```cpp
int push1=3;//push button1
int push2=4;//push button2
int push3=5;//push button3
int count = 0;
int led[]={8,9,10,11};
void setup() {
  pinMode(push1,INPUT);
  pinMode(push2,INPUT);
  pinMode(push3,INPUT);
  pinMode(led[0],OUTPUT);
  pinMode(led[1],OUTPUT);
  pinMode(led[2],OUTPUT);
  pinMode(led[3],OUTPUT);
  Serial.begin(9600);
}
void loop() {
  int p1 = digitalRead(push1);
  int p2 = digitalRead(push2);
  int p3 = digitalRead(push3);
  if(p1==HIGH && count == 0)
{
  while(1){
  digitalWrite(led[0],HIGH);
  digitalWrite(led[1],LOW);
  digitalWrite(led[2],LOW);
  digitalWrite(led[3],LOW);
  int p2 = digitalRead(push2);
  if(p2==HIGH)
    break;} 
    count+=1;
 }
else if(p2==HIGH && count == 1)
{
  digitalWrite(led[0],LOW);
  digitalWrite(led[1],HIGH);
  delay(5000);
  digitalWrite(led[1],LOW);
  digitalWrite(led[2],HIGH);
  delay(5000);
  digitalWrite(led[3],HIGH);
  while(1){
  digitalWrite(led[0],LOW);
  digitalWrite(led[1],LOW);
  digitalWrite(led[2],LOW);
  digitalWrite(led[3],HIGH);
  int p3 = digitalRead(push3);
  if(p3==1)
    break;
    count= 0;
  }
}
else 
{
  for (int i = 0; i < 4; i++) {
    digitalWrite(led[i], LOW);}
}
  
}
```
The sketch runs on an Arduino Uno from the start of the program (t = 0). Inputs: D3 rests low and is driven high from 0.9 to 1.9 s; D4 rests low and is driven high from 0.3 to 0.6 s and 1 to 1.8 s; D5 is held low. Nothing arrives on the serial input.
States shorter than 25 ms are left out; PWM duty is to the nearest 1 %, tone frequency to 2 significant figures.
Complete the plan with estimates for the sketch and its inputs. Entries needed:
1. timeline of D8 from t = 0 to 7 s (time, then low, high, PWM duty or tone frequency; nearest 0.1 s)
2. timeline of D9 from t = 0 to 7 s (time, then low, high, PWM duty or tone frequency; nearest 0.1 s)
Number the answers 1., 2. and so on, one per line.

1. 0 s low; 0.9 s high; 1 s low
2. 0 s low; 1 s high; 6 s low
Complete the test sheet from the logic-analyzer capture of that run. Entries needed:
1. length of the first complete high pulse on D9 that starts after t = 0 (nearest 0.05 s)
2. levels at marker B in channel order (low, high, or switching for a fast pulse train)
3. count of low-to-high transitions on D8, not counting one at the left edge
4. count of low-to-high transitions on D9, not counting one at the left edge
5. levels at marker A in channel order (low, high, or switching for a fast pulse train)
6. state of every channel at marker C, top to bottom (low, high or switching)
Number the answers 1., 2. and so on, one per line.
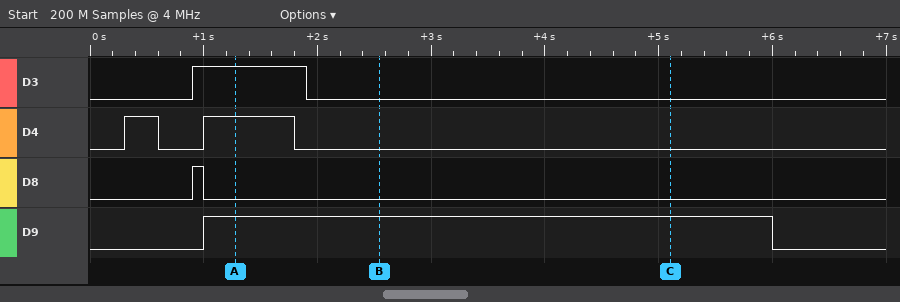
1. 5.00 s
2. D3 low, D4 low, D8 low, D9 high
3. 1
4. 1
5. D3 high, D4 high, D8 low, D9 high
6. D3 low, D4 low, D8 low, D9 high
